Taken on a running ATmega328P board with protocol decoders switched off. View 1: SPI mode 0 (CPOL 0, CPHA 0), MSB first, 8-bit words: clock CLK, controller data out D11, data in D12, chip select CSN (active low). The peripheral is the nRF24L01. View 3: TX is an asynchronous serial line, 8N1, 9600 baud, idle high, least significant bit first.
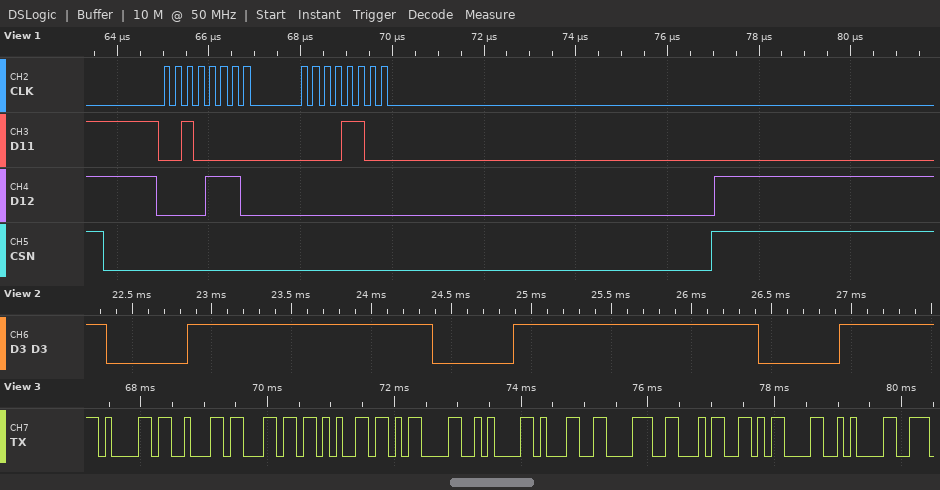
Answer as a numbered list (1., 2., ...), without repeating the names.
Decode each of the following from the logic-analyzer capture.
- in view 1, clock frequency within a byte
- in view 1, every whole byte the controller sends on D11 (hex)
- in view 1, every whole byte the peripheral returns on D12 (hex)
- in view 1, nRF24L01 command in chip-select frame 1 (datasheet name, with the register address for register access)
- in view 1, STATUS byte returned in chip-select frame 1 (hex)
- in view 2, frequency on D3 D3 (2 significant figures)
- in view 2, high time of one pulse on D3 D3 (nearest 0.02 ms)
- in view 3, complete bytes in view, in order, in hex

1. 4 MHz
2. 0x20 0x0C
3. 0x0E 0x00
4. W_REGISTER 0x00
5. 0x0E
6. 490 Hz
7. 1.54 ms
8. 61 62 6C 65 0D 0A 31 38 34 0D 0A
